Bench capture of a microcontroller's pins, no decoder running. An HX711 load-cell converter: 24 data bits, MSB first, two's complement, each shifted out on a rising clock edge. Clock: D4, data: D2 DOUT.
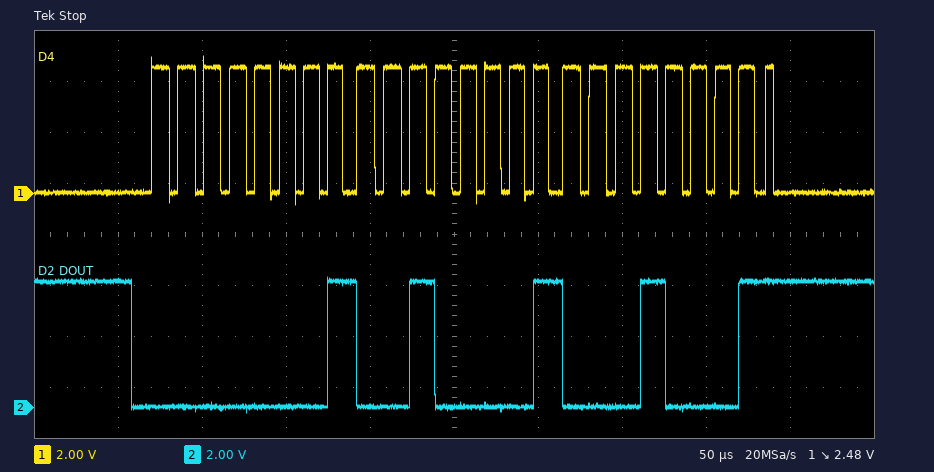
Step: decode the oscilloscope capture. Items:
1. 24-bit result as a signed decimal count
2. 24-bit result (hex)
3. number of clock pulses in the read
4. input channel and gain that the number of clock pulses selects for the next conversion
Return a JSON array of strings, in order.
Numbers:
["74001", "0x012111", "25", "channel A, gain 128"]
